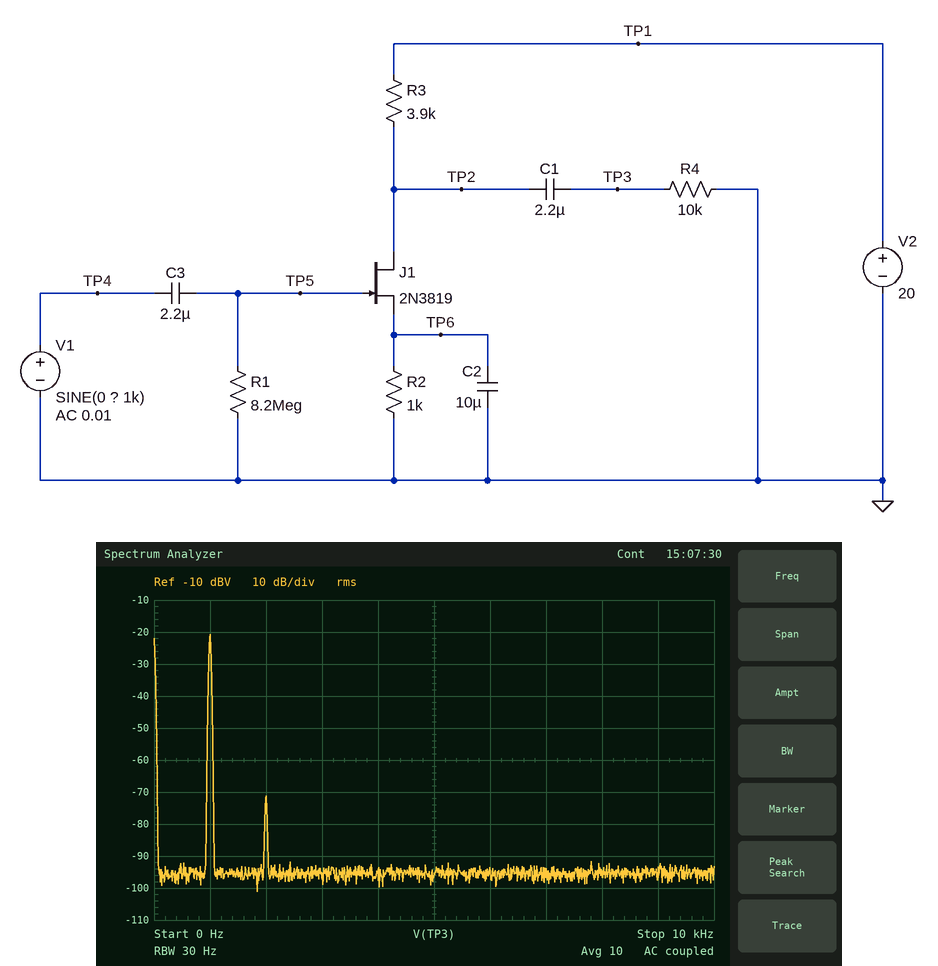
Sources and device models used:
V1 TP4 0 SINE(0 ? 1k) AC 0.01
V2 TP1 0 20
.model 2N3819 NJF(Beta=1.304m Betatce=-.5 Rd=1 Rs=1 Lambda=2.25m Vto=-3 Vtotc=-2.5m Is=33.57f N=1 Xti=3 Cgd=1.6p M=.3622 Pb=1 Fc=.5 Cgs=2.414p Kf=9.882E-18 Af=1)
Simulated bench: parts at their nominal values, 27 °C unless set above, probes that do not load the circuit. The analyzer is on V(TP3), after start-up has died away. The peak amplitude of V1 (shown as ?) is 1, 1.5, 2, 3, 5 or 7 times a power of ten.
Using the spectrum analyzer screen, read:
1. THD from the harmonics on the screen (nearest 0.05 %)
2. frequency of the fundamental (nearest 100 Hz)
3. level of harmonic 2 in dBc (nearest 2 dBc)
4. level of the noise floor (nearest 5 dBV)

0.30 %
1.0 kHz
-50 dBc
-95 dBV
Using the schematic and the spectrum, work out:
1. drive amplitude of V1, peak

15 mV
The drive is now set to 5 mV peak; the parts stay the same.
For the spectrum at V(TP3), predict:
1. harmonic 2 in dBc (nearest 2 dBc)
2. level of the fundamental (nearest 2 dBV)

-60 dBc
-30 dBV
